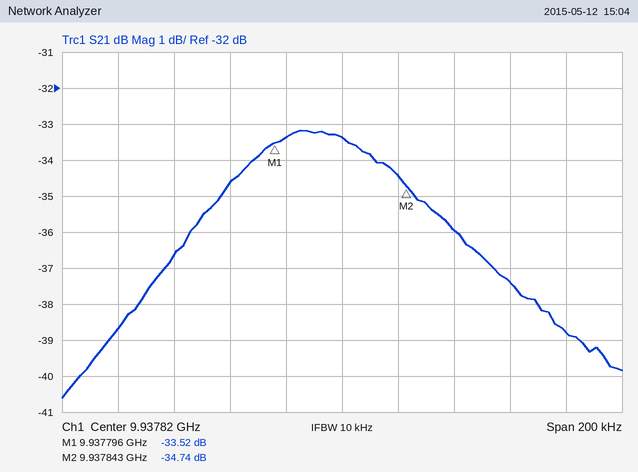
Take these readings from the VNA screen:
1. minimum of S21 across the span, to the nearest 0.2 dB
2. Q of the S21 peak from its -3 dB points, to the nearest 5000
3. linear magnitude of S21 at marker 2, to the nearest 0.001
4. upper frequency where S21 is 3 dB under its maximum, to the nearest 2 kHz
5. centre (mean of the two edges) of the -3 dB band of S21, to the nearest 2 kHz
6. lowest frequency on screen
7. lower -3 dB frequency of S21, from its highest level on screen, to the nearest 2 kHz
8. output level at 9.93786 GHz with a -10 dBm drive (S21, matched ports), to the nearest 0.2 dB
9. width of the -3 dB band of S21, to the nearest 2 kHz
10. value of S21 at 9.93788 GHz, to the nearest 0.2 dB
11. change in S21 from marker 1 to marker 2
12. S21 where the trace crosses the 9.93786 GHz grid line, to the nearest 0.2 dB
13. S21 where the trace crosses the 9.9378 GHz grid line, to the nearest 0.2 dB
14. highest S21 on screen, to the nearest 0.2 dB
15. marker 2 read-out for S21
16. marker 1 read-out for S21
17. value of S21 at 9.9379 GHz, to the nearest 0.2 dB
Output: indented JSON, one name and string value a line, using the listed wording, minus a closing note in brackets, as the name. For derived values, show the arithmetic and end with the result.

{
  "minimum of S21 across the span, to the nearest 0.2 dB": "-40.6 dB",
  "Q of the S21 peak from its -3 dB points, to the nearest 5000": "9.93781 GHz / 98 kHz ≈ 101406, so 100000 to the nearest 5000",
  "linear magnitude of S21 at marker 2, to the nearest 0.001": "10^(-34.74/20) ≈ 0.018",
  "upper frequency where S21 is 3 dB under its maximum, to the nearest 2 kHz": "9.937862 GHz",
  "centre (mean of the two edges) of the -3 dB band of S21, to the nearest 2 kHz": "9.937814 GHz",
  "lowest frequency on screen": "9.93772 GHz",
  "lower -3 dB frequency of S21, from its highest level on screen, to the nearest 2 kHz": "9.937764 GHz",
  "output level at 9.93786 GHz with a -10 dBm drive (S21, matched ports), to the nearest 0.2 dB": "-10 dBm + (-36.0 dB) = -46.0 dBm",
  "width of the -3 dB band of S21, to the nearest 2 kHz": "9.937862 GHz − 9.937764 GHz = 98 kHz",
  "value of S21 at 9.93788 GHz, to the nearest 0.2 dB": "-37.4 dB",
  "change in S21 from marker 1 to marker 2": "-34.74 − (-33.52) = -1.22 dB",
  "S21 where the trace crosses the 9.93786 GHz grid line, to the nearest 0.2 dB": "-36.0 dB",
  "S21 where the trace crosses the 9.9378 GHz grid line, to the nearest 0.2 dB": "-33.4 dB",
  "highest S21 on screen, to the nearest 0.2 dB": "-33.2 dB",
  "marker 2 read-out for S21": "-34.74 dB",
  "marker 1 read-out for S21": "-33.52 dB",
  "value of S21 at 9.9379 GHz, to the nearest 0.2 dB": "-38.8 dB"
}
